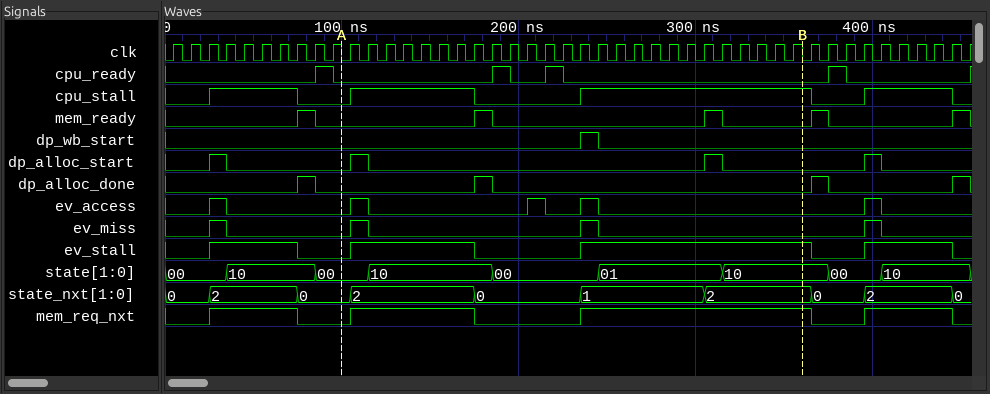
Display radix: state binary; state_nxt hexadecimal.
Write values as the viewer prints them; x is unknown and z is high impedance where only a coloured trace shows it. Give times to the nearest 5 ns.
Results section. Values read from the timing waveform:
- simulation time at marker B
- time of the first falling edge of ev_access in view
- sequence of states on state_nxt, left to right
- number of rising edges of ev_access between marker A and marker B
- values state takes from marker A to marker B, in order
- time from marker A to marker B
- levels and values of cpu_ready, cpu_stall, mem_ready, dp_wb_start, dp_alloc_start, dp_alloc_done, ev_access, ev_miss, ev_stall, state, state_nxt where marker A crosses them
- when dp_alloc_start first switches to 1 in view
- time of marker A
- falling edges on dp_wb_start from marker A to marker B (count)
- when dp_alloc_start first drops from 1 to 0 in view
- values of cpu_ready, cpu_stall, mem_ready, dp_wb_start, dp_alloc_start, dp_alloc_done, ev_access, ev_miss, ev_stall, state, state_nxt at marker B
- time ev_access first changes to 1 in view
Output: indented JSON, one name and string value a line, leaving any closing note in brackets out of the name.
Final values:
{
  "simulation time at marker B": "360 ns",
  "time of the first falling edge of ev_access in view": "35 ns",
  "sequence of states on state_nxt, left to right": "0, 2, 0, 2, 0, 1, 2, 0, 2, 0",
  "number of rising edges of ev_access between marker A and marker B": "3",
  "values state takes from marker A to marker B, in order": "00, 10, 00, 01, 10",
  "time from marker A to marker B": "260 ns",
  "levels and values of cpu_ready, cpu_stall, mem_ready, dp_wb_start, dp_alloc_start, dp_alloc_done, ev_access, ev_miss, ev_stall, state, state_nxt where marker A crosses them": "cpu_ready=0, cpu_stall=0, mem_ready=0, dp_wb_start=0, dp_alloc_start=0, dp_alloc_done=0, ev_access=0, ev_miss=0, ev_stall=0, state=00, state_nxt=0",
  "when dp_alloc_start first switches to 1 in view": "25 ns",
  "time of marker A": "100 ns",
  "falling edges on dp_wb_start from marker A to marker B": "1",
  "when dp_alloc_start first drops from 1 to 0 in view": "35 ns",
  "values of cpu_ready, cpu_stall, mem_ready, dp_wb_start, dp_alloc_start, dp_alloc_done, ev_access, ev_miss, ev_stall, state, state_nxt at marker B": "cpu_ready=0, cpu_stall=1, mem_ready=0, dp_wb_start=0, dp_alloc_start=0, dp_alloc_done=0, ev_access=0, ev_miss=0, ev_stall=1, state=10, state_nxt=2",
  "time ev_access first changes to 1 in view": "25 ns"
}
